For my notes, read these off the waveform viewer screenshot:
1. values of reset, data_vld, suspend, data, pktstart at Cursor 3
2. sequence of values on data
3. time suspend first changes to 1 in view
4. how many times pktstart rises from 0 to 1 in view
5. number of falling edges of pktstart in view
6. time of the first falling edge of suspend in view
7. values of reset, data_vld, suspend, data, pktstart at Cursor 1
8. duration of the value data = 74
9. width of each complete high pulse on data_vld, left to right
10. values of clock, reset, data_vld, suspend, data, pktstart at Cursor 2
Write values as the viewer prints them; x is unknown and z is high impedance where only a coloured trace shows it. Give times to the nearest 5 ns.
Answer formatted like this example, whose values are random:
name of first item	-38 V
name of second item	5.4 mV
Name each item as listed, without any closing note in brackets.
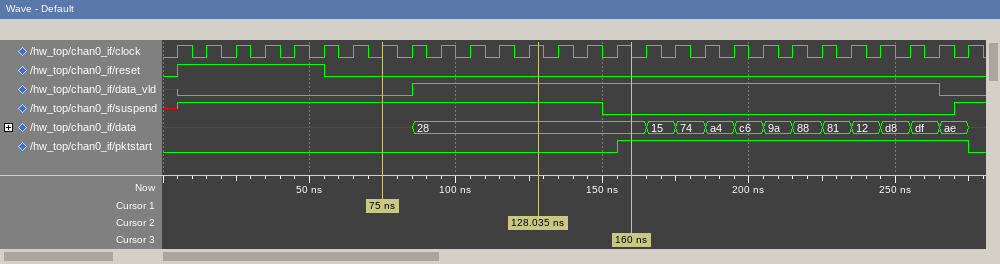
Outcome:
values of reset, data_vld, suspend, data, pktstart at Cursor 3	reset=0, data_vld=1, suspend=0, data=28, pktstart=1
sequence of values on data	x, 28, 15, 74, a4, c6, 9a, 88, 81, 12, d8, df, ae, x
time suspend first changes to 1 in view	5 ns
how many times pktstart rises from 0 to 1 in view	1
number of falling edges of pktstart in view	1
time of the first falling edge of suspend in view	150 ns
values of reset, data_vld, suspend, data, pktstart at Cursor 1	reset=0, data_vld=0, suspend=1, data=x, pktstart=0
duration of the value data = 74	10 ns
width of each complete high pulse on data_vld, left to right	180 ns
values of clock, reset, data_vld, suspend, data, pktstart at Cursor 2	clock=1, reset=0, data_vld=1, suspend=1, data=28, pktstart=0
